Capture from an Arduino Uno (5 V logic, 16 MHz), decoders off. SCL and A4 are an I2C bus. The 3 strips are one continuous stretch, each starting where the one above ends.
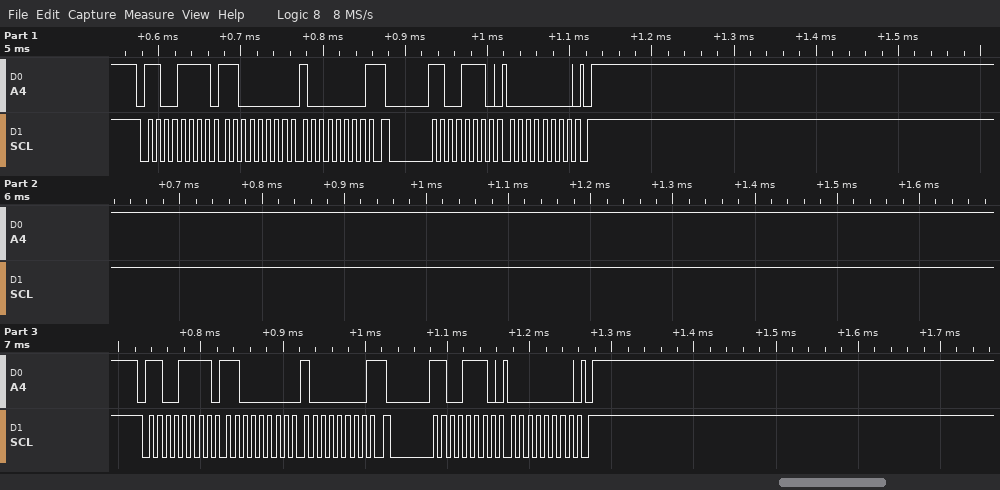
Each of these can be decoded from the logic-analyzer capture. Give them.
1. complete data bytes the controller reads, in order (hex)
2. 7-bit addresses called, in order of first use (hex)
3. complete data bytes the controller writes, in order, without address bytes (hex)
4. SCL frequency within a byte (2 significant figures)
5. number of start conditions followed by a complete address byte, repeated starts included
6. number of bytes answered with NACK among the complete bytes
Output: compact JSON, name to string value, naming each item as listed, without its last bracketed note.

{"complete data bytes the controller reads, in order": "C0 80 C0 80", "7-bit addresses called, in order of first use": "0x67", "complete data bytes the controller writes, in order, without address bytes": "00 00", "SCL frequency within a byte": "100 kHz", "number of start conditions followed by a complete address byte, repeated starts included": "4", "number of bytes answered with NACK among the complete bytes": "2"}
